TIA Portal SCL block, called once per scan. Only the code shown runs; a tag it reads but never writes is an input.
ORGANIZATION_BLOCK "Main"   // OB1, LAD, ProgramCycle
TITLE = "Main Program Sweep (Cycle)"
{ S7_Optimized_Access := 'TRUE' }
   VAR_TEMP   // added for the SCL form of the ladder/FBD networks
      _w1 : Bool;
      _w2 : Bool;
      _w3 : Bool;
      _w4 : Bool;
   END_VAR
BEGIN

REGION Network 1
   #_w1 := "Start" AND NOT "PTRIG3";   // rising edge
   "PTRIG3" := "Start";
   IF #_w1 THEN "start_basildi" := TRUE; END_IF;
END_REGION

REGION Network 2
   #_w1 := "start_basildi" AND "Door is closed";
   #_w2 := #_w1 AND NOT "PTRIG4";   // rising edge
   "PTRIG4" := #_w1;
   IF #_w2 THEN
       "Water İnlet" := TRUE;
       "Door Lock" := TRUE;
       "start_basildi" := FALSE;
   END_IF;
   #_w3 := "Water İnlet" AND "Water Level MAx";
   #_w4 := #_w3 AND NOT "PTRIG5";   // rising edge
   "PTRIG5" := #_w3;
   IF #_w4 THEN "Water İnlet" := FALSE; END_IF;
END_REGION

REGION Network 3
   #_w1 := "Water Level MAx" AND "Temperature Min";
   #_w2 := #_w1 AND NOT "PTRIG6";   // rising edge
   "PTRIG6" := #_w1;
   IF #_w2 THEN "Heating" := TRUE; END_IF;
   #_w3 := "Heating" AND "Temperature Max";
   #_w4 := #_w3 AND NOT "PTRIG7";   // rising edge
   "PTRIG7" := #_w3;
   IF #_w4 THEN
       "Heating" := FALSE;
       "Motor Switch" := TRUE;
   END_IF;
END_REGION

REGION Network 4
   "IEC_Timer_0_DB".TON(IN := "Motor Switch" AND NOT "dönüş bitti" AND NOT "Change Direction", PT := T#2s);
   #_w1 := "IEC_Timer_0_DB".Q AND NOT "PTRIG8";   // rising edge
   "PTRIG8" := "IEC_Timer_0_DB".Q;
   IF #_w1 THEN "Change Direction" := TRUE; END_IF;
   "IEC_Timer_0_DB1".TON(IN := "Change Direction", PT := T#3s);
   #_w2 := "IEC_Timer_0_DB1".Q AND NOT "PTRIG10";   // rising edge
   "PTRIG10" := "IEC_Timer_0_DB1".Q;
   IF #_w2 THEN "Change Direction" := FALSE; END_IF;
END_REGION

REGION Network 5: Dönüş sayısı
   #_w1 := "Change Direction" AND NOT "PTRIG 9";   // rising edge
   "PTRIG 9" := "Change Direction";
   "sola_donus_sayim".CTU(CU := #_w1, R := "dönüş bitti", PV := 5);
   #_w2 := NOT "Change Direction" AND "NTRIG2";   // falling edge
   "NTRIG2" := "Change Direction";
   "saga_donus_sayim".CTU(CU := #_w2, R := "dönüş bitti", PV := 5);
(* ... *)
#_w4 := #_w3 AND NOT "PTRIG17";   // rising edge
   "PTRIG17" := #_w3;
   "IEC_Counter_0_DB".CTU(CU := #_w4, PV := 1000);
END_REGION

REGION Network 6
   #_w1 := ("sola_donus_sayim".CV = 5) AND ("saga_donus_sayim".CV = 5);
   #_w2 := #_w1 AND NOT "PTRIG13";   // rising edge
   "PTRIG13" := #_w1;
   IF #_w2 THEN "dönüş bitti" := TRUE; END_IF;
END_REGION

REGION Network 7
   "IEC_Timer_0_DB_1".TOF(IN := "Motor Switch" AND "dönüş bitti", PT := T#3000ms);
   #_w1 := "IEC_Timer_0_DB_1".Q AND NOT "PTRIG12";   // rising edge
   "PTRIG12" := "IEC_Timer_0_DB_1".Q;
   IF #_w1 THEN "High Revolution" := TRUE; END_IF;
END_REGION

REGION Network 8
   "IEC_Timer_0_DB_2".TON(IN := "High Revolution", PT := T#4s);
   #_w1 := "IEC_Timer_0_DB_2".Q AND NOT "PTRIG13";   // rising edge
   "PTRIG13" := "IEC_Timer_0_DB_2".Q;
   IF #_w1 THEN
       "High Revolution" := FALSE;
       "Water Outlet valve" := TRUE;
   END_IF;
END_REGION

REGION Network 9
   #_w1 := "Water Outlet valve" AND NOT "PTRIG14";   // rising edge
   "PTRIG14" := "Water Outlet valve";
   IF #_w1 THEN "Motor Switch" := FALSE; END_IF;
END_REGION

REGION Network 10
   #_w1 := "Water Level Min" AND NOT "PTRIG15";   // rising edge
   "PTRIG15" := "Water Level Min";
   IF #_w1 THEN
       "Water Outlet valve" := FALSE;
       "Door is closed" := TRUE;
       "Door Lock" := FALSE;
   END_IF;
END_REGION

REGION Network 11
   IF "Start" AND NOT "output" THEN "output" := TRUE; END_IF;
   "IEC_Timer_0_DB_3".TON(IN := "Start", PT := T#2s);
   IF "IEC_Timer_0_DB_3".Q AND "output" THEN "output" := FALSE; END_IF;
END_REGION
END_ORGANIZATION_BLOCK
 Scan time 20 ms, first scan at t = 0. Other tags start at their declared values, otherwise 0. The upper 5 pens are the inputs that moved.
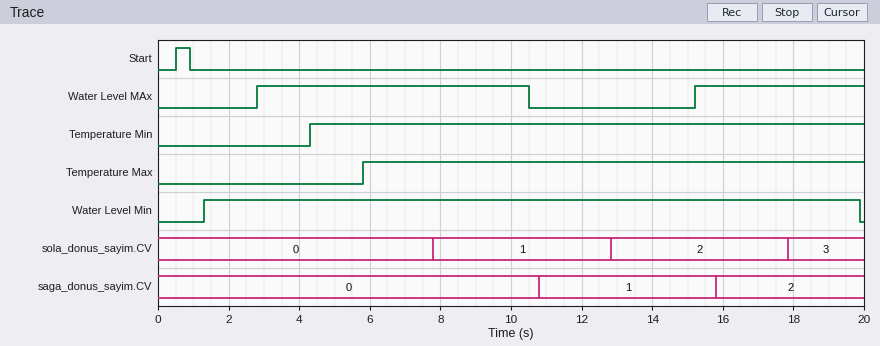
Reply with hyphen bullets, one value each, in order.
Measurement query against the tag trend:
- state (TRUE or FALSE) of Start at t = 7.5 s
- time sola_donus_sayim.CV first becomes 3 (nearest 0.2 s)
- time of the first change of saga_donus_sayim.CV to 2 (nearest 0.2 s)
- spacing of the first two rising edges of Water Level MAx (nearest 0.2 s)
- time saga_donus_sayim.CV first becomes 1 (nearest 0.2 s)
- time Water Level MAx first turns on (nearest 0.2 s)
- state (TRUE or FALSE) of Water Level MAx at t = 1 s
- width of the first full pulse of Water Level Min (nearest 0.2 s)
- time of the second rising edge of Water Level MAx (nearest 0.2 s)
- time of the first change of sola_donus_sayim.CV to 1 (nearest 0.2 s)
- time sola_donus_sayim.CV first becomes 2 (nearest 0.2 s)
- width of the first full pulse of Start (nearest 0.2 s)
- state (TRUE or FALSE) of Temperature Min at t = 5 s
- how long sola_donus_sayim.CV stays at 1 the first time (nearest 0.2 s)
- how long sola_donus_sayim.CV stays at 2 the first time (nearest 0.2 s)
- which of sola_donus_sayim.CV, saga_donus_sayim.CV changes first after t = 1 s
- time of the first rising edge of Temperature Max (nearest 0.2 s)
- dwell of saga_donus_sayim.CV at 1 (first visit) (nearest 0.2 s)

- FALSE
- 17.8 s
- 15.8 s
- 12.4 s
- 10.8 s
- 2.8 s
- FALSE
- 18.6 s
- 15.2 s
- 7.8 s
- 12.8 s
- 0.4 s
- TRUE
- 5.0 s
- 5.0 s
- sola_donus_sayim.CV
- 5.8 s
- 5.0 s
